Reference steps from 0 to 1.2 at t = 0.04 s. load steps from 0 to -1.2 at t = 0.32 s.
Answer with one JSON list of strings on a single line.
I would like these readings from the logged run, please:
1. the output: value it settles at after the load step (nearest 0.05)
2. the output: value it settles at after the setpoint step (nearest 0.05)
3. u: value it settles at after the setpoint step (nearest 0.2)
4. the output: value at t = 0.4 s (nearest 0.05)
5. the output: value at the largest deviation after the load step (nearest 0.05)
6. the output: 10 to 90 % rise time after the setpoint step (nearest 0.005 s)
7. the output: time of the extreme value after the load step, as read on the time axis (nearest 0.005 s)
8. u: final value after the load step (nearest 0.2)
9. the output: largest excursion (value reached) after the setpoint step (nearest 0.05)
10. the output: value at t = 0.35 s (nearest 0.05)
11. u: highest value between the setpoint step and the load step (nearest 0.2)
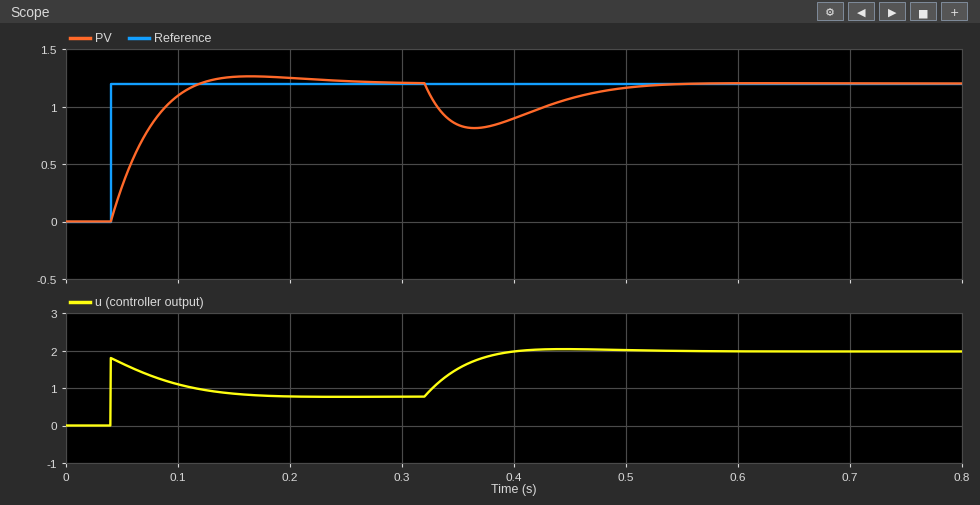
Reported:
["1.20", "1.20", "0.8", "0.90", "0.80", "0.055 s", "0.365 s", "2.0", "1.25", "0.85", "1.8"]
